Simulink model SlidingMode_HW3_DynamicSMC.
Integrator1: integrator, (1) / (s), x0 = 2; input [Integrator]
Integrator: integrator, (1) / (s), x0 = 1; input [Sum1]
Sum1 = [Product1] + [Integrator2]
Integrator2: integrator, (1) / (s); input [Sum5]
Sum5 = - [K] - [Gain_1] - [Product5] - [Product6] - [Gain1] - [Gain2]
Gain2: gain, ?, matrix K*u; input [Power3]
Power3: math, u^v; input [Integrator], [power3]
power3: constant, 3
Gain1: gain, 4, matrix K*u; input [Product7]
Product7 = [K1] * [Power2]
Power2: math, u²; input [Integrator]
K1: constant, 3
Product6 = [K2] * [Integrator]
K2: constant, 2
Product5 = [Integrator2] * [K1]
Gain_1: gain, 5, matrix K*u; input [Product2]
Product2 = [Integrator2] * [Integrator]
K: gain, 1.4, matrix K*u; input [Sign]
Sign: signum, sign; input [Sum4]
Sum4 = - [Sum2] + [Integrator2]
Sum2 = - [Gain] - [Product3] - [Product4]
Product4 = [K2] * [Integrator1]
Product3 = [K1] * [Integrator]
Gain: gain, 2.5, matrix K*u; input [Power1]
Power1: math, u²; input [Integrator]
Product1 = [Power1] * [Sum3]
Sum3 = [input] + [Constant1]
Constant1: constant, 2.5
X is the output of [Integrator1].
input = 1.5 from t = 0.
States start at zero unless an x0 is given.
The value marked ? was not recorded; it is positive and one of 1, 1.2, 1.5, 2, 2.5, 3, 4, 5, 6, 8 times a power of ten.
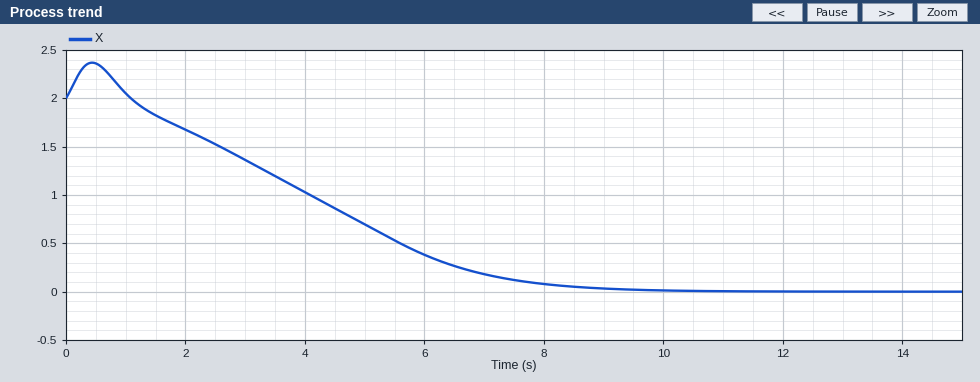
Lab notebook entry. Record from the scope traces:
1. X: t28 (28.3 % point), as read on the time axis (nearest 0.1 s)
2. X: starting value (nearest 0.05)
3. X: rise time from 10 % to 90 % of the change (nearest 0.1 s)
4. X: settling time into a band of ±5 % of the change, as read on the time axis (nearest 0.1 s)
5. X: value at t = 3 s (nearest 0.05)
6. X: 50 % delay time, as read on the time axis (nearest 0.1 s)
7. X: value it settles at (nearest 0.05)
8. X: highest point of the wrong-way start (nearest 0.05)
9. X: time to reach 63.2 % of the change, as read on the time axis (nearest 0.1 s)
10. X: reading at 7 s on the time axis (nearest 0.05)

2.8 s
2.00
5.3 s
7.8 s
1.35
4.1 s
0.00
2.35
4.9 s
0.20
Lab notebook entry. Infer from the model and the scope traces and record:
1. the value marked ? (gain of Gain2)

40
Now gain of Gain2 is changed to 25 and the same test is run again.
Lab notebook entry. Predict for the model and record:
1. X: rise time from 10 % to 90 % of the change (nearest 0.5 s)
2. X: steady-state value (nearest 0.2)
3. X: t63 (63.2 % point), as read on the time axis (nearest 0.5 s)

4.0 s
0.0
4.5 s
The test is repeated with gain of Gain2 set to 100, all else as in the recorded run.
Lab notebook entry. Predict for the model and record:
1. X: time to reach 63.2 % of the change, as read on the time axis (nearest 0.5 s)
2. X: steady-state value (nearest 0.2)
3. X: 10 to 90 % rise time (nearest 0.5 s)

7.0 s
0.0
7.0 s
